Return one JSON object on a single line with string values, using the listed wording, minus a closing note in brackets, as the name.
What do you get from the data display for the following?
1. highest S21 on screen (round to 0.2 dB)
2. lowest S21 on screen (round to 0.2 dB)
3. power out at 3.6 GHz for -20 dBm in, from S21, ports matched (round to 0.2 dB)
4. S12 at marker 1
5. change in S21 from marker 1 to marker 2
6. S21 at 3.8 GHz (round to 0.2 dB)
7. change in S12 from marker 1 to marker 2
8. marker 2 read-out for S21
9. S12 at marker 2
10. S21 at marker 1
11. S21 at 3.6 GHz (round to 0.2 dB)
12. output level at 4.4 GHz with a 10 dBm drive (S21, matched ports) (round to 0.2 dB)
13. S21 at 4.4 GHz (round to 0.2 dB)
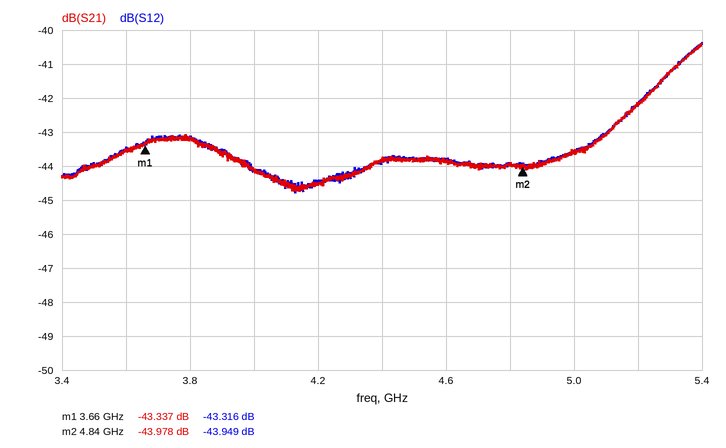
{"highest S21 on screen": "-40.4 dB", "lowest S21 on screen": "-44.8 dB", "power out at 3.6 GHz for -20 dBm in, from S21, ports matched": "-63.6 dBm", "S12 at marker 1": "-43.316 dB", "change in S21 from marker 1 to marker 2": "-0.641 dB", "S21 at 3.8 GHz": "-43.2 dB", "change in S12 from marker 1 to marker 2": "-0.633 dB", "marker 2 read-out for S21": "-43.978 dB", "S12 at marker 2": "-43.949 dB", "S21 at marker 1": "-43.337 dB", "S21 at 3.6 GHz": "-43.6 dB", "output level at 4.4 GHz with a 10 dBm drive (S21, matched ports)": "-33.8 dBm", "S21 at 4.4 GHz": "-43.8 dB"}
